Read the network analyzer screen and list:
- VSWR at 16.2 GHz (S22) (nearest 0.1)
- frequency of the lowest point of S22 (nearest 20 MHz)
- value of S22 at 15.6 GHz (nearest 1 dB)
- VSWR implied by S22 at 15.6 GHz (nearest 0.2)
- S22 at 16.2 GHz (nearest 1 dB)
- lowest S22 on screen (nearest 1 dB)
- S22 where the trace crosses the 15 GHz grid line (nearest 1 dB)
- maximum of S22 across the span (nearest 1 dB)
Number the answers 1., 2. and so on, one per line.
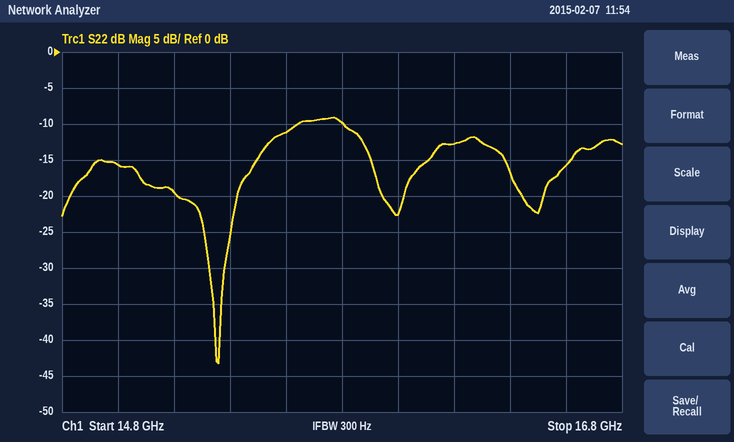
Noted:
1. 1.6
2. 15.36 GHz
3. -11 dB
4. 1.8
5. -13 dB
6. -43 dB
7. -16 dB
8. -9 dB
